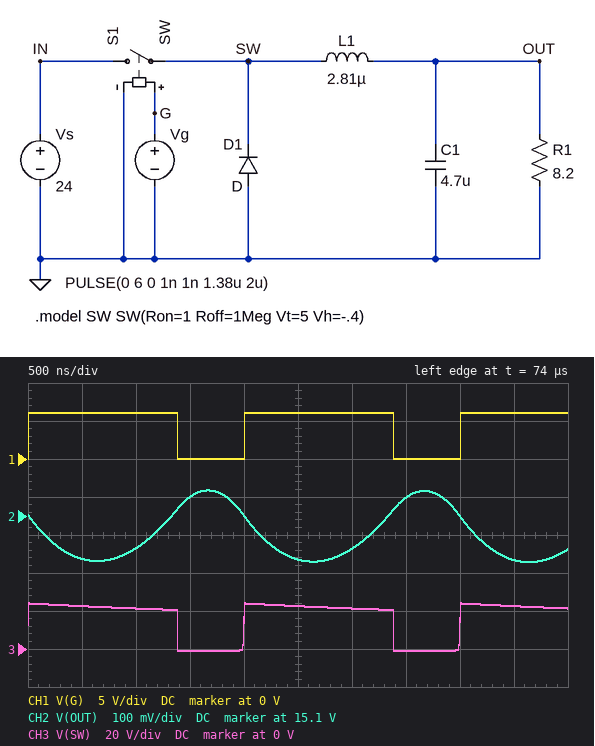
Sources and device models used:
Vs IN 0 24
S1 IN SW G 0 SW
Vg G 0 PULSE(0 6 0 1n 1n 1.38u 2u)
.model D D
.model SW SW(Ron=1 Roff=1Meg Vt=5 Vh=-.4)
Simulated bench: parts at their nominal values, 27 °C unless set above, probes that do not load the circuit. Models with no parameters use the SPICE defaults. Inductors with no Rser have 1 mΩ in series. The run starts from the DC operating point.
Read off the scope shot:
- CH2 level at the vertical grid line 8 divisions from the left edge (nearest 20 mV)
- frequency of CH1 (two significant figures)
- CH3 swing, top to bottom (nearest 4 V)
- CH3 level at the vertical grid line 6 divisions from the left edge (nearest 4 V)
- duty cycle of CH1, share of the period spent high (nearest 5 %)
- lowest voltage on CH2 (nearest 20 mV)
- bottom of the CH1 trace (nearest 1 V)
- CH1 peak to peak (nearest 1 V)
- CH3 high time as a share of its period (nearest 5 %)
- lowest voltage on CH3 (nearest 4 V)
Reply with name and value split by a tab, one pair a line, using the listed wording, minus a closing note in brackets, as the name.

CH2 level at the vertical grid line 8 divisions from the left edge	15.10 V
frequency of CH1	500 kHz
CH3 swing, top to bottom	24 V
CH3 level at the vertical grid line 6 divisions from the left edge	20 V
duty cycle of CH1, share of the period spent high	70 %
lowest voltage on CH2	14.98 V
bottom of the CH1 trace	0 V
CH1 peak to peak	6 V
CH3 high time as a share of its period	70 %
lowest voltage on CH3	0 V
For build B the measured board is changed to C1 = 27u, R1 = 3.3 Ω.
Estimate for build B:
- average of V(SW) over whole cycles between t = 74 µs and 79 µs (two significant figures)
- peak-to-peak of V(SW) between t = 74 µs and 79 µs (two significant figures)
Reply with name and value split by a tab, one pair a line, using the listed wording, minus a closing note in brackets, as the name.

average of V(SW) over whole cycles between t = 74 µs and 79 µs	13 V
peak-to-peak of V(SW) between t = 74 µs and 79 µs	22 V
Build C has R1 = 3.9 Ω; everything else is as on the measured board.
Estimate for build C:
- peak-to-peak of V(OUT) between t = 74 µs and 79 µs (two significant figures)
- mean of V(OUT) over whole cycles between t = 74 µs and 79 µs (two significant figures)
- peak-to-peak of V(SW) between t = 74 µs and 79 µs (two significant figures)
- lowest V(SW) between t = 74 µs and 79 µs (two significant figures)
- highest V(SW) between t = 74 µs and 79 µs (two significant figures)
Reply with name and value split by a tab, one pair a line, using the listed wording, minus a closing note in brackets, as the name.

peak-to-peak of V(OUT) between t = 74 µs and 79 µs	170 mV
mean of V(OUT) over whole cycles between t = 74 µs and 79 µs	14 V
peak-to-peak of V(SW) between t = 74 µs and 79 µs	23 V
lowest V(SW) between t = 74 µs and 79 µs	-880 mV
highest V(SW) between t = 74 µs and 79 µs	22 V
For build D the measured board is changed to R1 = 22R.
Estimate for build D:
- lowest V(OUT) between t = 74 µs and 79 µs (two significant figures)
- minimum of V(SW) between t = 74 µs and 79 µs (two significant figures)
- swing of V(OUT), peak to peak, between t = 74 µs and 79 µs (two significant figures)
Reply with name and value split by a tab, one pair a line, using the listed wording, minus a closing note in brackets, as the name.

lowest V(OUT) between t = 74 µs and 79 µs	19 V
minimum of V(SW) between t = 74 µs and 79 µs	-850 mV
swing of V(OUT), peak to peak, between t = 74 µs and 79 µs	120 mV
